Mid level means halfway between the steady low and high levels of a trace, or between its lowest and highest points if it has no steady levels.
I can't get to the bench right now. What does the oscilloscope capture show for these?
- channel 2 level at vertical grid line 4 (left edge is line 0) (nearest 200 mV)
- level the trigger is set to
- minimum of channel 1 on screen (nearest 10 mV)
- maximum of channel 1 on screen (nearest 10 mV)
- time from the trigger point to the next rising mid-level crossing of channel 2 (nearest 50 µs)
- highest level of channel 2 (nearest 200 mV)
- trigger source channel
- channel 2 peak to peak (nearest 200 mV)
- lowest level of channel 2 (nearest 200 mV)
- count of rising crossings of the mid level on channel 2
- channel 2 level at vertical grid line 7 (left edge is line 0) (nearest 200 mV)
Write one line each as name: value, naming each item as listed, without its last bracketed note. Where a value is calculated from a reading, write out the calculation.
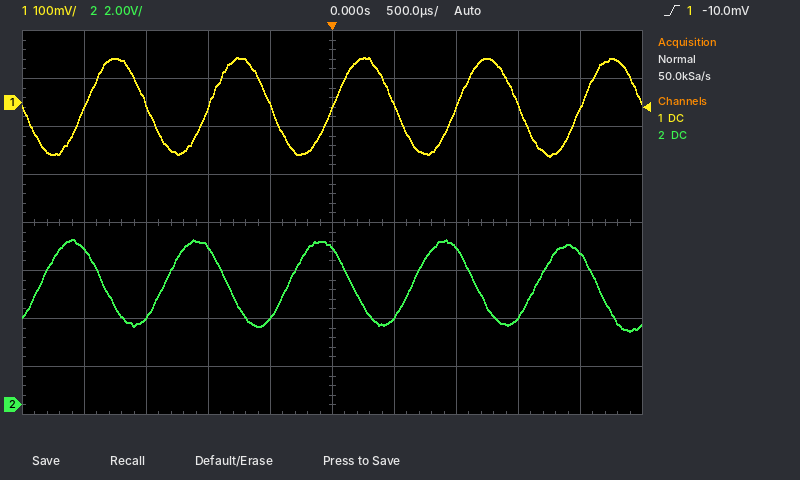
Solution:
channel 2 level at vertical grid line 4 (left edge is line 0): 3.6 V
level the trigger is set to: -10.0 mV
minimum of channel 1 on screen: -110 mV
maximum of channel 1 on screen: 90 mV
time from the trigger point to the next rising mid-level crossing of channel 2: 650 µs
highest level of channel 2: 6.8 V
trigger source channel: channel 1
channel 2 peak to peak: 6.8 V − (3.0 V) = 3.8 V
lowest level of channel 2: 3.0 V
count of rising crossings of the mid level on channel 2: 5
channel 2 level at vertical grid line 7 (left edge is line 0): 6.6 V
